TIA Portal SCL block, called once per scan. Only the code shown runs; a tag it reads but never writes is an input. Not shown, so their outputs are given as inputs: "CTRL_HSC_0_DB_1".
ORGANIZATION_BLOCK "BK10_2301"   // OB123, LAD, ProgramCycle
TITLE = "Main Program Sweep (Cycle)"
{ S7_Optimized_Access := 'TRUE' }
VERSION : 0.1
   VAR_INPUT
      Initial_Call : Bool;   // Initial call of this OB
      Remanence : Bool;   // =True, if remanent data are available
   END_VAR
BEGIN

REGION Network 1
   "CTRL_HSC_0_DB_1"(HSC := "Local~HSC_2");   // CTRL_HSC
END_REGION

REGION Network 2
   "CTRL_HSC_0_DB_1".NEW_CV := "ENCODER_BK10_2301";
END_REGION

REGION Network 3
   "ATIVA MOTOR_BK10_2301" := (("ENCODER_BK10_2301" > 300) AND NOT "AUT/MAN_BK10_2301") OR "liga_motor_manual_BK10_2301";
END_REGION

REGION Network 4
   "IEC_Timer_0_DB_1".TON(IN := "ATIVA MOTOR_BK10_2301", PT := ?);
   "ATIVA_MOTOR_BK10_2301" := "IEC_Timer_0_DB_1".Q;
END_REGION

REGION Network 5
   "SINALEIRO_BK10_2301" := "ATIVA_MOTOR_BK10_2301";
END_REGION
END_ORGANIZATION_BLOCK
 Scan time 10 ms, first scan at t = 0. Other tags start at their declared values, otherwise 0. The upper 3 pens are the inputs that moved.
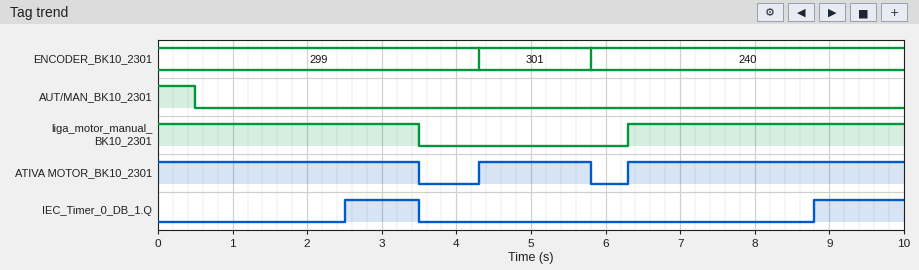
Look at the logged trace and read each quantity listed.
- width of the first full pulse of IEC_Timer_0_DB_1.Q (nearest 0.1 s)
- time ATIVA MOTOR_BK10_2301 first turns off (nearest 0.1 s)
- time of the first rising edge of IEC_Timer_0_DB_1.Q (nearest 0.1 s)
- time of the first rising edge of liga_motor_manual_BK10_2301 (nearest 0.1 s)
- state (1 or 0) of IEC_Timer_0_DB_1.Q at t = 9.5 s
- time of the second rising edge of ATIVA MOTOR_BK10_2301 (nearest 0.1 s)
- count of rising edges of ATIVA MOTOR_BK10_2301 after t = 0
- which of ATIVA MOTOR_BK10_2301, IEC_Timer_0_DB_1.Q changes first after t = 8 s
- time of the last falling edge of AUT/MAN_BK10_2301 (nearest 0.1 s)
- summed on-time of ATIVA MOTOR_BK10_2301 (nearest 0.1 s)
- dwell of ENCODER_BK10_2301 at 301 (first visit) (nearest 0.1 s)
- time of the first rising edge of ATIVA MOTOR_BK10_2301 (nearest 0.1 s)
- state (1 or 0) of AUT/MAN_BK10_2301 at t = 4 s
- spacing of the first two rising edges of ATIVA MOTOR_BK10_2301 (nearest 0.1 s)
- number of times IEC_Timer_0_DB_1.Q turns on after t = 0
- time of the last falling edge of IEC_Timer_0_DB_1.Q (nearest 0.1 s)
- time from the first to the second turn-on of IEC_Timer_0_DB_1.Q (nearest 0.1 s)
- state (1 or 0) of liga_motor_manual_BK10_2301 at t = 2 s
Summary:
1.0 s
3.5 s
2.5 s
6.3 s
1
6.3 s
2
IEC_Timer_0_DB_1.Q
0.5 s
8.7 s
1.5 s
4.3 s
0
2.0 s
2
3.5 s
6.3 s
1
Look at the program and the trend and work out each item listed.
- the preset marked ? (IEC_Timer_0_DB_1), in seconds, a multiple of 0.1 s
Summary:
2.5 s
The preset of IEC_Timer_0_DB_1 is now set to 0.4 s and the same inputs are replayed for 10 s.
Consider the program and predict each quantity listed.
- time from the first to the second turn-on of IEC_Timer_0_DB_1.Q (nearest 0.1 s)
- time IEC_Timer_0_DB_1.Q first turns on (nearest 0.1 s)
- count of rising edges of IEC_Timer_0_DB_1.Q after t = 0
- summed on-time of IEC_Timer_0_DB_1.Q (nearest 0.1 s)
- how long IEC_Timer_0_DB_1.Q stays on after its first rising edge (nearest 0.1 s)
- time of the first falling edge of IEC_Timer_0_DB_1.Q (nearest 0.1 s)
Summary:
4.3 s
0.4 s
3
7.5 s
3.1 s
3.5 s
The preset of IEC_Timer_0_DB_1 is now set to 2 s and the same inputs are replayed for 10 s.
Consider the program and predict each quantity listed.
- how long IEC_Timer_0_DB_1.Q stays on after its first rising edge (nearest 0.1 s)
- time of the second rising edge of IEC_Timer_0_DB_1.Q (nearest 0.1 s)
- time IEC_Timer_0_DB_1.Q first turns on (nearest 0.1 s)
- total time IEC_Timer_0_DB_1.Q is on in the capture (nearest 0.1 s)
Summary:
1.5 s
8.3 s
2.0 s
3.2 s
